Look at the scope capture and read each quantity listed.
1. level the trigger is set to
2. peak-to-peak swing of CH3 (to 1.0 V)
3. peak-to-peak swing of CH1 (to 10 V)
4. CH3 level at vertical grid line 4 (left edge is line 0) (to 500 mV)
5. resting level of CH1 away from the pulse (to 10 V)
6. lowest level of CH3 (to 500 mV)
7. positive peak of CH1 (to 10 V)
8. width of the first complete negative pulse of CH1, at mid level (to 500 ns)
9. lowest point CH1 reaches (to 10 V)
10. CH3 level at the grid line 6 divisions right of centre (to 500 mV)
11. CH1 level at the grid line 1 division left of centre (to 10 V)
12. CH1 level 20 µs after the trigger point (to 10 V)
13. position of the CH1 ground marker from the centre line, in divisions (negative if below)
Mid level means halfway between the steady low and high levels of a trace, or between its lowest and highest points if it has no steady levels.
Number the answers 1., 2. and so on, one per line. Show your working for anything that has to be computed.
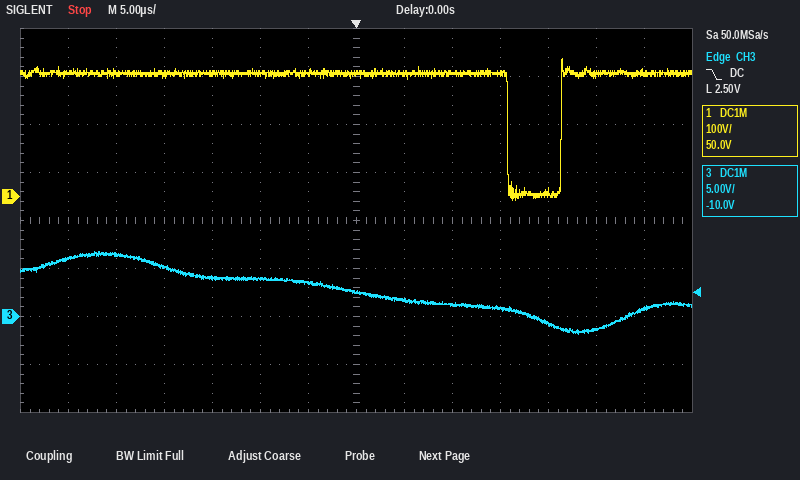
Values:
1. 2.50 V
2. 9.0 V
3. 290 V − (-10 V) = 300 V
4. 4.0 V
5. 260 V
6. -2.0 V
7. 290 V
8. 5.5 µs
9. -10 V
10. 1.0 V
11. 260 V
12. 10 V
13. +0.5 div
